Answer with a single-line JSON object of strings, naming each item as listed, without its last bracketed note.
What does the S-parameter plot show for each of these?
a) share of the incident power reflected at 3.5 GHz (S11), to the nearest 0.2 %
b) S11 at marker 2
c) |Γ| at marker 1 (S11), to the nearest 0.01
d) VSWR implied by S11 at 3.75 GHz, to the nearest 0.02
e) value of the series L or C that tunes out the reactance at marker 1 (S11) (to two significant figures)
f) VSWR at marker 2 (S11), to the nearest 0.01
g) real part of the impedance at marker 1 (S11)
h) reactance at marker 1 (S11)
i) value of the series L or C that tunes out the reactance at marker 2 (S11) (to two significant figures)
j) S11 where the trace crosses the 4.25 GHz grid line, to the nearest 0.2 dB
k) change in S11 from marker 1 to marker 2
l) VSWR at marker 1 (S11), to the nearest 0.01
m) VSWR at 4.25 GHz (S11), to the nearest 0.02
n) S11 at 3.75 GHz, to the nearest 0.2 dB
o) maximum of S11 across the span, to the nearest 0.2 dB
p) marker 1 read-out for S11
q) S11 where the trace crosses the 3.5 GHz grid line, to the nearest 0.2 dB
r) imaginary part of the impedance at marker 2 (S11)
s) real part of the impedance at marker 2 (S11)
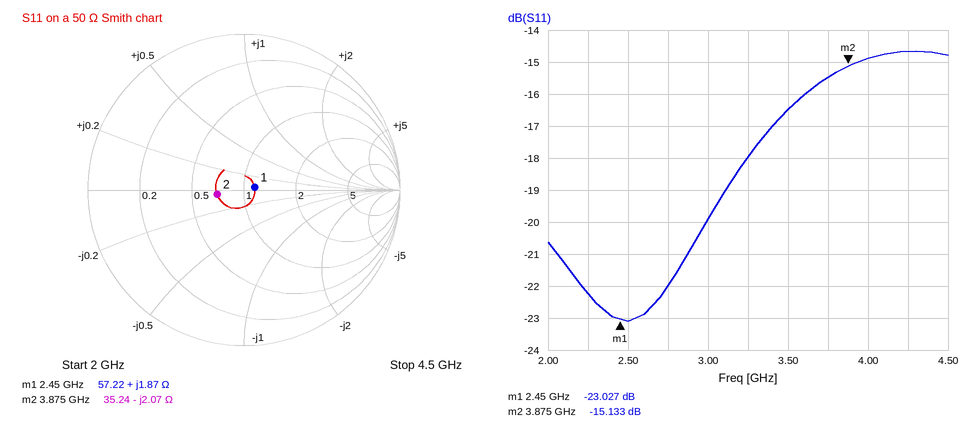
{"share of the incident power reflected at 3.5 GHz (S11), to the nearest 0.2 %": "2.2 %", "S11 at marker 2": "-15.133 dB", "|Γ| at marker 1 (S11), to the nearest 0.01": "0.07", "VSWR implied by S11 at 3.75 GHz, to the nearest 0.02": "1.40", "value of the series L or C that tunes out the reactance at marker 1 (S11)": "35 pF", "VSWR at marker 2 (S11), to the nearest 0.01": "1.42", "real part of the impedance at marker 1": "57.22 Ω", "reactance at marker 1": "+1.87 Ω", "value of the series L or C that tunes out the reactance at marker 2 (S11)": "85 pH", "S11 where the trace crosses the 4.25 GHz grid line, to the nearest 0.2 dB": "-14.6 dB", "change in S11 from marker 1 to marker 2": "7.894 dB", "VSWR at marker 1 (S11), to the nearest 0.01": "1.15", "VSWR at 4.25 GHz (S11), to the nearest 0.02": "1.46", "S11 at 3.75 GHz, to the nearest 0.2 dB": "-15.4 dB", "maximum of S11 across the span, to the nearest 0.2 dB": "-14.6 dB", "marker 1 read-out for S11": "-23.027 dB", "S11 where the trace crosses the 3.5 GHz grid line, to the nearest 0.2 dB": "-16.4 dB", "imaginary part of the impedance at marker 2": "-2.07 Ω", "real part of the impedance at marker 2": "35.24 Ω"}
